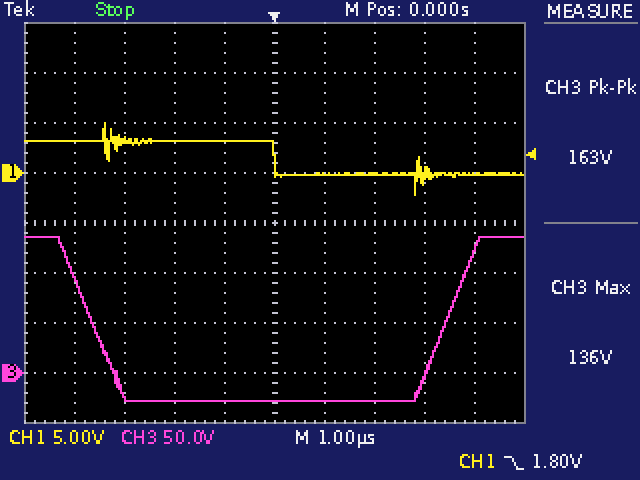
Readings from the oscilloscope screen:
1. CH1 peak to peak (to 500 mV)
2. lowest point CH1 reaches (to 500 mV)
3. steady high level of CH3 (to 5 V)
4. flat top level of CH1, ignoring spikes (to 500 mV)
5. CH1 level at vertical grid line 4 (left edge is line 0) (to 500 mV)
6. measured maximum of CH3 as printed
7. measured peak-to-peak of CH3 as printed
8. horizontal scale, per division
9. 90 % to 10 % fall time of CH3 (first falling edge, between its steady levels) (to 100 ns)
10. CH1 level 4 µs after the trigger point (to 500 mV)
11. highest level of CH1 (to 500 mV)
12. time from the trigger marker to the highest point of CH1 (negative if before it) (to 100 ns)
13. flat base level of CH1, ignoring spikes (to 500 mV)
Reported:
7.0 V
-2.0 V
135 V
3.0 V
3.0 V
136 V
163 V
1 µs
1.1 µs
0.0 V
5.0 V
-3.4 µs
0.0 V
